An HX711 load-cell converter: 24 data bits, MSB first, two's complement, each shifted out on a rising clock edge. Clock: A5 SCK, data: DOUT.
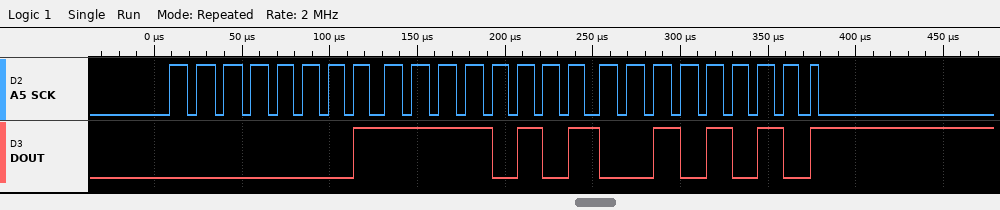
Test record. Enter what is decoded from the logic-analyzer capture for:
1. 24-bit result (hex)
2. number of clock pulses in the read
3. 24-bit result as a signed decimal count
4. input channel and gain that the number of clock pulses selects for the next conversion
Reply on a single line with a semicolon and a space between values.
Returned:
0x01F52A; 25; 128298; channel A, gain 128
